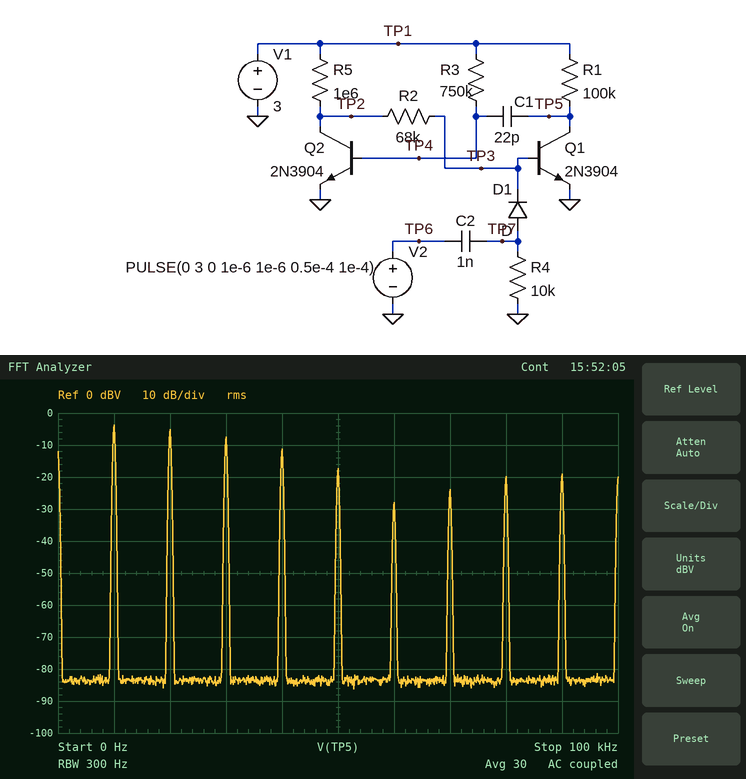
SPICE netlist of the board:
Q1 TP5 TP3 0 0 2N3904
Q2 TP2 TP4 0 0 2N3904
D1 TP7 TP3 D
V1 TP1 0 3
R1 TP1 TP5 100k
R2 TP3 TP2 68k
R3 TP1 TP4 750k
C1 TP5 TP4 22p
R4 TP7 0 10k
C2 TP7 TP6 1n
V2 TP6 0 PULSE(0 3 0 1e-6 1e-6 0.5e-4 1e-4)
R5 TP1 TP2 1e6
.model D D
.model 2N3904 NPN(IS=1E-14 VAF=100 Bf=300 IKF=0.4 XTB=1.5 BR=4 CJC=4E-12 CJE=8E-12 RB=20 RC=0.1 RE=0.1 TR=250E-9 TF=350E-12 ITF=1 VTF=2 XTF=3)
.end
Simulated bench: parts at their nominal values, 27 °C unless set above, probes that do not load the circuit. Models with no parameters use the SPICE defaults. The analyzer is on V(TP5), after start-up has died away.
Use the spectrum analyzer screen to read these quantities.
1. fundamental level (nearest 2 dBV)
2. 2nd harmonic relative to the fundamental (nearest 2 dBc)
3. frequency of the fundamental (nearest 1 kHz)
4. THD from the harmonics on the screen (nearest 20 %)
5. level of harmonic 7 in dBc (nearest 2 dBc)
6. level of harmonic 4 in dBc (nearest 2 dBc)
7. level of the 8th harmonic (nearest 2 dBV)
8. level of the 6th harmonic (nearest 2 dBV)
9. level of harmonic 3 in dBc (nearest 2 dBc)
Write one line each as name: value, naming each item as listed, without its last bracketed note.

fundamental level: -4 dBV
2nd harmonic relative to the fundamental: -2 dBc
frequency of the fundamental: 10 kHz
THD from the harmonics on the screen: 120 %
level of harmonic 7 in dBc: -20 dBc
level of harmonic 4 in dBc: -8 dBc
level of the 8th harmonic: -20 dBV
level of the 6th harmonic: -28 dBV
level of harmonic 3 in dBc: -4 dBc
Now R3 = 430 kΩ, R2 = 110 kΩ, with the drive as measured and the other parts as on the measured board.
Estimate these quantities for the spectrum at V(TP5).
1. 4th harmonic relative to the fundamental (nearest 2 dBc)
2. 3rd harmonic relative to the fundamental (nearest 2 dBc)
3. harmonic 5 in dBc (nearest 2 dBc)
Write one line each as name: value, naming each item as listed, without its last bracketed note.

4th harmonic relative to the fundamental: -4 dBc
3rd harmonic relative to the fundamental: -2 dBc
harmonic 5 in dBc: -6 dBc
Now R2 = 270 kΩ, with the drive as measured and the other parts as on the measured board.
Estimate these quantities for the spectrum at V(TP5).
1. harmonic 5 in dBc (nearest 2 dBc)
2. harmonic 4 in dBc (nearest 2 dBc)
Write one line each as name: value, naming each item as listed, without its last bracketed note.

harmonic 5 in dBc: -18 dBc
harmonic 4 in dBc: -10 dBc
